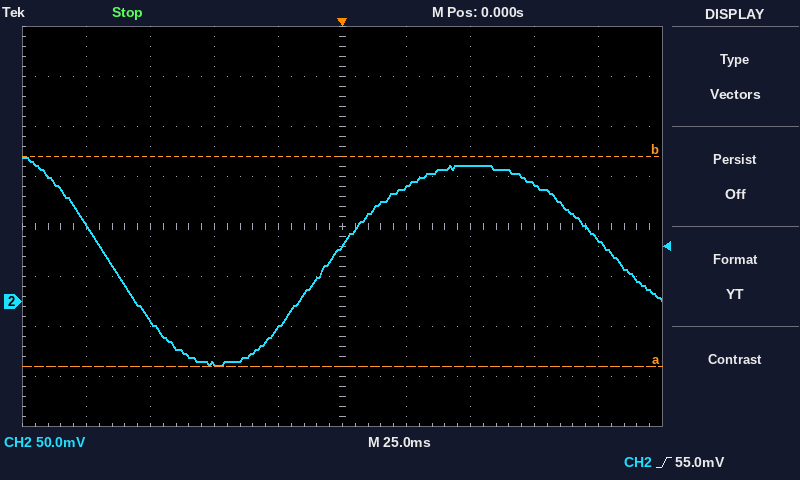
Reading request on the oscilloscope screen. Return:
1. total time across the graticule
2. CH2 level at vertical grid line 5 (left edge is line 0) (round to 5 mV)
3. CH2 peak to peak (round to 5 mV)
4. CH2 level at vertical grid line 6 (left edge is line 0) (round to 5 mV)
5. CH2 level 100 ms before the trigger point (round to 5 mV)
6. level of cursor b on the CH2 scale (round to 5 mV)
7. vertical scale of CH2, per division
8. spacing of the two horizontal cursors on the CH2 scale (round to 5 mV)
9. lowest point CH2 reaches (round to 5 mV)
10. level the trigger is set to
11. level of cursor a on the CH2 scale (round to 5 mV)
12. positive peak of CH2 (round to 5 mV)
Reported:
250 ms
55 mV
210 mV
115 mV
75 mV
145 mV
50 mV
210 mV
-65 mV
55.0 mV
-65 mV
145 mV
